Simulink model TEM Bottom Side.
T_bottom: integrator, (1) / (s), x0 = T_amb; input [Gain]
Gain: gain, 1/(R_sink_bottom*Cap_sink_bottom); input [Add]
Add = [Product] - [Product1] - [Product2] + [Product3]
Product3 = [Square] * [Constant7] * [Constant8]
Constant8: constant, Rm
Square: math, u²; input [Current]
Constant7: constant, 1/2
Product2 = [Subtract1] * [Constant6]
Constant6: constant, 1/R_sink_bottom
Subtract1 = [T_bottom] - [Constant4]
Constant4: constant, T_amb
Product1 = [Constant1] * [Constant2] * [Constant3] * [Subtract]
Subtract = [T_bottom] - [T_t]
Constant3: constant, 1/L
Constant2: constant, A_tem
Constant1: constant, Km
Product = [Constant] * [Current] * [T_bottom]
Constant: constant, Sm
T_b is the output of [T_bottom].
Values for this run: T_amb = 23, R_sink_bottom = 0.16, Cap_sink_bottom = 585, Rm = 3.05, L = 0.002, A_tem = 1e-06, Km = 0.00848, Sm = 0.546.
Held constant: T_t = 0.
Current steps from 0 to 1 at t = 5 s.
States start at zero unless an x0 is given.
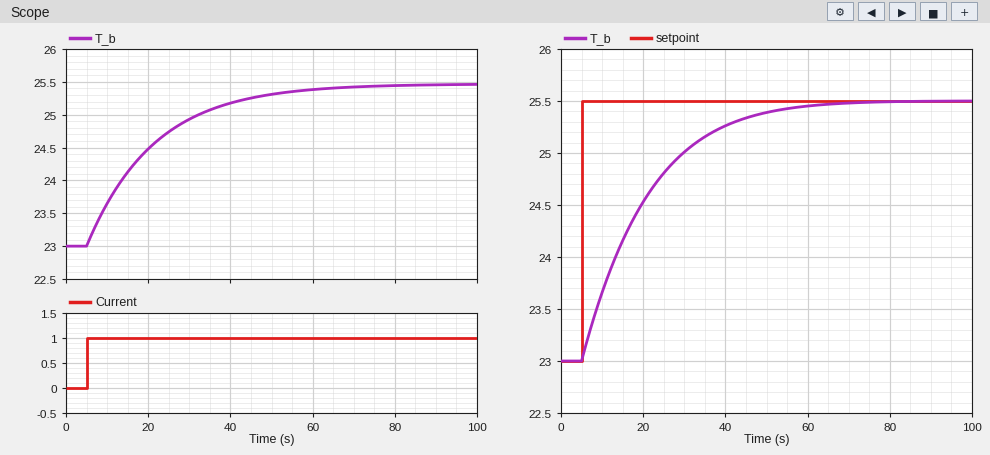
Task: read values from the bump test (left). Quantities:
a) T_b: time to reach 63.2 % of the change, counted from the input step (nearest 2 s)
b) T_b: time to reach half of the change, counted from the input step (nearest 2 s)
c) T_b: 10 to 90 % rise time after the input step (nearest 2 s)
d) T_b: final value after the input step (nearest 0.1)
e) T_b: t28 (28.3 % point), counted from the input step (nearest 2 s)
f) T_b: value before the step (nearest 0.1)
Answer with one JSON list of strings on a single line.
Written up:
["16 s", "12 s", "36 s", "25.5", "6 s", "23.0"]
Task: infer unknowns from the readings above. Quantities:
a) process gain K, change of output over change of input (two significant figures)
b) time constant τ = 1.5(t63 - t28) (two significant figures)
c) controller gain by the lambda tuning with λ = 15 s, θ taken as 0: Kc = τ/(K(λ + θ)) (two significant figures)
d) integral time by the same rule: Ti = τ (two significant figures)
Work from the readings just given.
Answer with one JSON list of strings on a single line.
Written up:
["2.5", "15 s", "0.40", "15 s"]
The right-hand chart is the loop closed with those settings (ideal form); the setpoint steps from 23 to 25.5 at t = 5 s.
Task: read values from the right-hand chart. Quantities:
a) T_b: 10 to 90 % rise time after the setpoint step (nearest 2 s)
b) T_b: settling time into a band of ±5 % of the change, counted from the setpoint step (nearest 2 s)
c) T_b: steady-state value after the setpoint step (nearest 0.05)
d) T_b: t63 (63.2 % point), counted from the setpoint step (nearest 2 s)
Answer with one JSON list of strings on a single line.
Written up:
["32 s", "44 s", "25.50", "16 s"]
